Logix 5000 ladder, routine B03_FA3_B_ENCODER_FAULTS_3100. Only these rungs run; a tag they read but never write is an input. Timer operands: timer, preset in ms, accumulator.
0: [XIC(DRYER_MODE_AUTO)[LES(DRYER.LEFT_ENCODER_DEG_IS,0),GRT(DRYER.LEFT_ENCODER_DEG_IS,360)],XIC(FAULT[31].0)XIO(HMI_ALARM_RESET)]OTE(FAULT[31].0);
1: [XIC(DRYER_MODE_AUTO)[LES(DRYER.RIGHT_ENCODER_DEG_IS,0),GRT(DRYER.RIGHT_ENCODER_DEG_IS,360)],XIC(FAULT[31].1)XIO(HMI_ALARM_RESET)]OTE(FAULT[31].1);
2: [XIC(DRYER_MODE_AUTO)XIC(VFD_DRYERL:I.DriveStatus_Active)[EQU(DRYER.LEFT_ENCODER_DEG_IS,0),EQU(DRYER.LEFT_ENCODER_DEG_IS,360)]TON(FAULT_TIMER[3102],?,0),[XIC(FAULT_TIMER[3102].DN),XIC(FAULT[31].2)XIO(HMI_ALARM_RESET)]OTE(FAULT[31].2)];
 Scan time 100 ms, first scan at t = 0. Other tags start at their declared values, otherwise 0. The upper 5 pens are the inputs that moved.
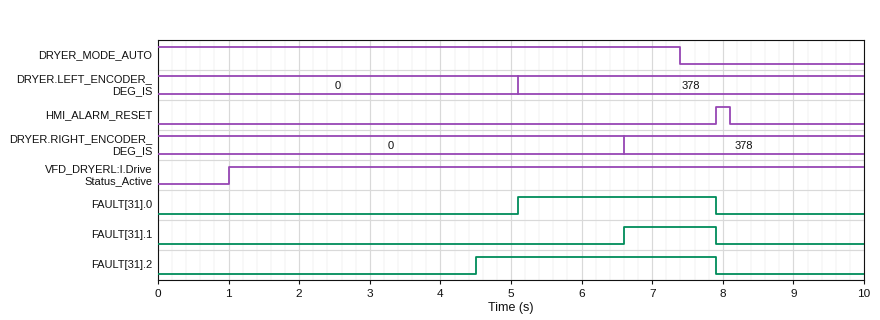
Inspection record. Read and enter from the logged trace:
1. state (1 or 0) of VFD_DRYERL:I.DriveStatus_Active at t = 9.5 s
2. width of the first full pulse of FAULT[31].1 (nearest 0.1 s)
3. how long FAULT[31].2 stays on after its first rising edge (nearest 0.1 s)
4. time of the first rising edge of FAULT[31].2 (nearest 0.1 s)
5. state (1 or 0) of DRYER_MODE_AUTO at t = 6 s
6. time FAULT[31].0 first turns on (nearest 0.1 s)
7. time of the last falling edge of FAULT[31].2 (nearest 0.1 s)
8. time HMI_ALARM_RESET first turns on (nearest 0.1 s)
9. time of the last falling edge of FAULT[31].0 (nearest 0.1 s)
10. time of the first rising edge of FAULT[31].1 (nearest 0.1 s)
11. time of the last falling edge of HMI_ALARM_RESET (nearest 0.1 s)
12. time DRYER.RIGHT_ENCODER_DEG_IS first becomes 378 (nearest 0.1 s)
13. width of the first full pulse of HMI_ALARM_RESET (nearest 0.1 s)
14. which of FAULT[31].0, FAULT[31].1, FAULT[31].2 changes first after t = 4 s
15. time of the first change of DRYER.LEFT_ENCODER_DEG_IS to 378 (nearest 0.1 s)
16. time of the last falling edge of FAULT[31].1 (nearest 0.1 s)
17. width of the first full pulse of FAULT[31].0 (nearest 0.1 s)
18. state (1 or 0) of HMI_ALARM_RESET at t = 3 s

1
1.3 s
3.4 s
4.5 s
1
5.1 s
7.9 s
7.9 s
7.9 s
6.6 s
8.1 s
6.6 s
0.2 s
FAULT[31].2
5.1 s
7.9 s
2.8 s
0
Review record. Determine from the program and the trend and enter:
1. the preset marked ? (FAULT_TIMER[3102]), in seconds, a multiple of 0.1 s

3.5 s
